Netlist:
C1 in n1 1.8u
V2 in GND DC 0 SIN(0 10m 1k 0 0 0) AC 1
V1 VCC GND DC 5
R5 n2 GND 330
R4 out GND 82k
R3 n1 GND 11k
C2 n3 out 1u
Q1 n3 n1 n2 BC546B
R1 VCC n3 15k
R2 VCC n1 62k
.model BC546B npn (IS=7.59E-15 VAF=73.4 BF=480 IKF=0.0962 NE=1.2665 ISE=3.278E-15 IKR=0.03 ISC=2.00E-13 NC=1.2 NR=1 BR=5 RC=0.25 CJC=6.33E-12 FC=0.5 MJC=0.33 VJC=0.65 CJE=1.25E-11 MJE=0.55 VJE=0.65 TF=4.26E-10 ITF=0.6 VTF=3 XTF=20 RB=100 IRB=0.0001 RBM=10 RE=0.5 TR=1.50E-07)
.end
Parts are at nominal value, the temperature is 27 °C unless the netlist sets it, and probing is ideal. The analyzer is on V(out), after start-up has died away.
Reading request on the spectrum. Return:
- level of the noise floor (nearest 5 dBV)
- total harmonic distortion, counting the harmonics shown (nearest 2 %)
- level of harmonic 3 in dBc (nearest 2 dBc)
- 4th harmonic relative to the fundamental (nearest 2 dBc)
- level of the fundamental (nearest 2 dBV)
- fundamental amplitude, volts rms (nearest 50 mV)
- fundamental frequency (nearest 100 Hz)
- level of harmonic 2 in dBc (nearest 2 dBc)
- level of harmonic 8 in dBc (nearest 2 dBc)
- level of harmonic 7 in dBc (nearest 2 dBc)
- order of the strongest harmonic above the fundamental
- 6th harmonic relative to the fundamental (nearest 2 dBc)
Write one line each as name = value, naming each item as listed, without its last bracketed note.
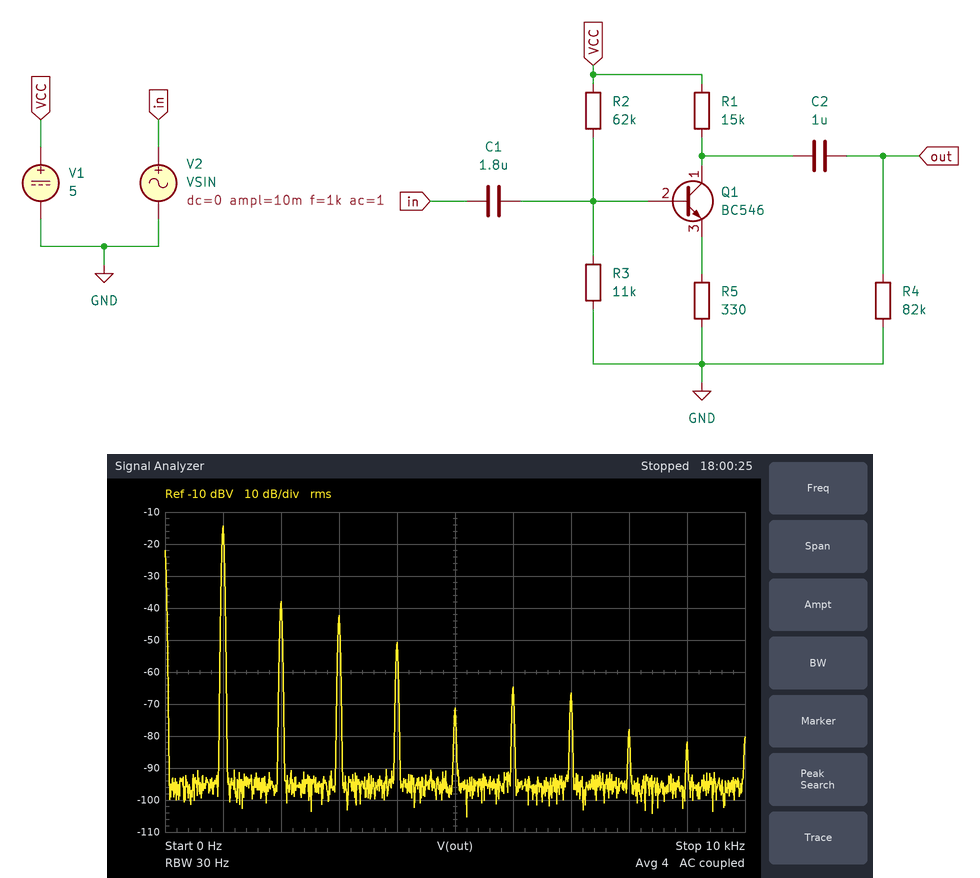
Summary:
level of the noise floor = -95 dBV
total harmonic distortion, counting the harmonics shown = 8 %
level of harmonic 3 in dBc = -28 dBc
4th harmonic relative to the fundamental = -36 dBc
level of the fundamental = -14 dBV
fundamental amplitude, volts rms = 200 mV
fundamental frequency = 1.0 kHz
level of harmonic 2 in dBc = -24 dBc
level of harmonic 8 in dBc = -64 dBc
level of harmonic 7 in dBc = -52 dBc
order of the strongest harmonic above the fundamental = 2
6th harmonic relative to the fundamental = -50 dBc
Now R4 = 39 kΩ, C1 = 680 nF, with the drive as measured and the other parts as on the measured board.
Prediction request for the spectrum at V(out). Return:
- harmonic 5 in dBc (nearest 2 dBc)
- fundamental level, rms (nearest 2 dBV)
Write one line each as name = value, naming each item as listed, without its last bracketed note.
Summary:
harmonic 5 in dBc = -54 dBc
fundamental level, rms = -16 dBV
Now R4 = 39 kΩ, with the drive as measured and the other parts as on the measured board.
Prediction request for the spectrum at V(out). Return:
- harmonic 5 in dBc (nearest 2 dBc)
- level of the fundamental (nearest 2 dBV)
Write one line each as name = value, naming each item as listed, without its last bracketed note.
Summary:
harmonic 5 in dBc = -56 dBc
level of the fundamental = -16 dBV
